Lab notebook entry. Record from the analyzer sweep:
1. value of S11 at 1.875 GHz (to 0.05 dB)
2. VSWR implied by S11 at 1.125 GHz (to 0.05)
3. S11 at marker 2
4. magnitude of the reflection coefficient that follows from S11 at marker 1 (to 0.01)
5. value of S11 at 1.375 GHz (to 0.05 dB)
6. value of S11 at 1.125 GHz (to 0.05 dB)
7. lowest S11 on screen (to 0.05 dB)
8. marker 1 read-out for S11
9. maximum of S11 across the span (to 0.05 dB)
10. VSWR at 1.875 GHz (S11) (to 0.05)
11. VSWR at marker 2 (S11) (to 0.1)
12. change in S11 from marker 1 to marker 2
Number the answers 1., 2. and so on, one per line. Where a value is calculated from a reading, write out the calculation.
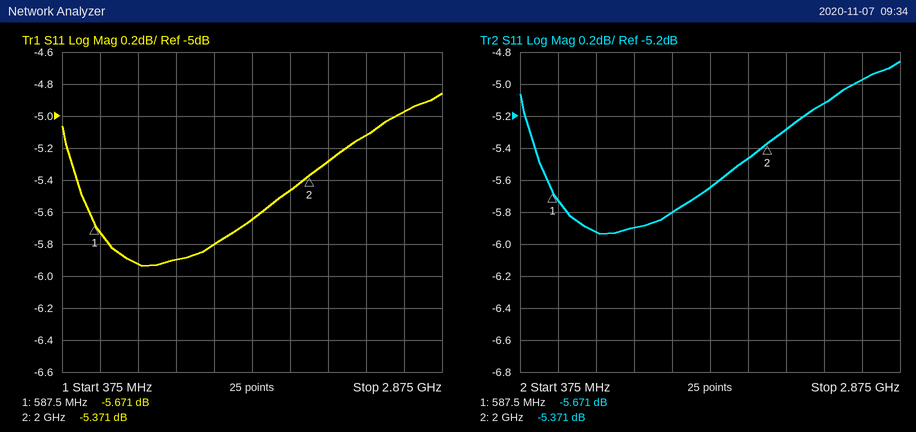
1. -5.45 dB
2. |Γ| = 10^(-5.9/20) = 0.5070; VSWR = (1 + 0.5070)/(1 − 0.5070) ≈ 3.06, so 3.05 to the nearest 0.05
3. -5.371 dB
4. 10^(-5.671/20) ≈ 0.52
5. -5.80 dB
6. -5.90 dB
7. -5.95 dB
8. -5.671 dB
9. -4.85 dB
10. |Γ| = 10^(-5.45/20) = 0.5339; VSWR = (1 + 0.5339)/(1 − 0.5339) ≈ 3.29, so 3.30 to the nearest 0.05
11. (1 + 0.5388)/(1 − 0.5388) ≈ 3.3
12. -5.371 − (-5.671) = 0.300 dB
